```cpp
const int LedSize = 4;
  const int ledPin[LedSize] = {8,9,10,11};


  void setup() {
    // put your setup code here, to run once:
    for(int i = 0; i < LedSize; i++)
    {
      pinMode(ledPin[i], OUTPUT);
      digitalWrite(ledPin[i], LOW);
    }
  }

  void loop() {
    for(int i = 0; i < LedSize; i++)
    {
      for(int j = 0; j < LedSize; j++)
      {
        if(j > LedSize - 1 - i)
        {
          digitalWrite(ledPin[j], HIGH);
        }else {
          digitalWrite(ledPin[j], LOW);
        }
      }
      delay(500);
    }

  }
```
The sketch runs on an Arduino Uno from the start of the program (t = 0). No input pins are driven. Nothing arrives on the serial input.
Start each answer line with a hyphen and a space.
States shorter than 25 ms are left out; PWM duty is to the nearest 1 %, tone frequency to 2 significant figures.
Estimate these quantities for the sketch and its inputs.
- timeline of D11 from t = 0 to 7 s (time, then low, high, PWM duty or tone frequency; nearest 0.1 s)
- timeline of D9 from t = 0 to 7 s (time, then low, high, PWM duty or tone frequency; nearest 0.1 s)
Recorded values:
- 0 s low; 0.5 s high; 2 s low; 2.5 s high; 4 s low; 4.5 s high; 6 s low; 6.5 s high
- 0 s low; 1.5 s high; 2 s low; 3.5 s high; 4 s low; 5.5 s high; 6 s low
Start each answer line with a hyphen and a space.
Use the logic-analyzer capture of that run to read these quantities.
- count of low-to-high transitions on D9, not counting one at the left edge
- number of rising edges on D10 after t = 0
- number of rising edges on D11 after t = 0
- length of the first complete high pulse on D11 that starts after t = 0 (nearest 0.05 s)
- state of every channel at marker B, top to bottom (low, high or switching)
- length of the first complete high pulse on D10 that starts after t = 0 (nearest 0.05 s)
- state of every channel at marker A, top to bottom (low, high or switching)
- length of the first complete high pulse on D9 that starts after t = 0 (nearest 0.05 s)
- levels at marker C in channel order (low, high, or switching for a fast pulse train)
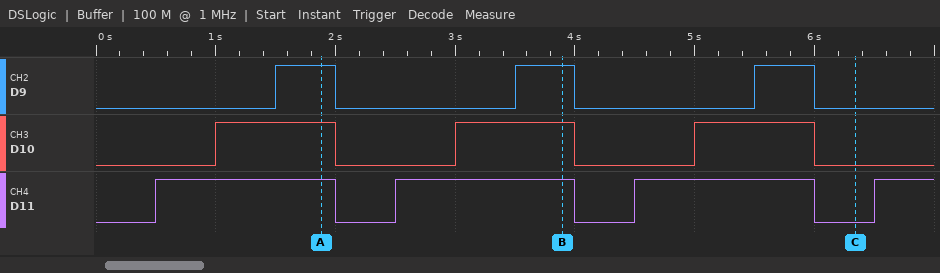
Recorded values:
- 3
- 3
- 4
- 1.50 s
- D9 high, D10 high, D11 high
- 1.00 s
- D9 high, D10 high, D11 high
- 0.50 s
- D9 low, D10 low, D11 low
